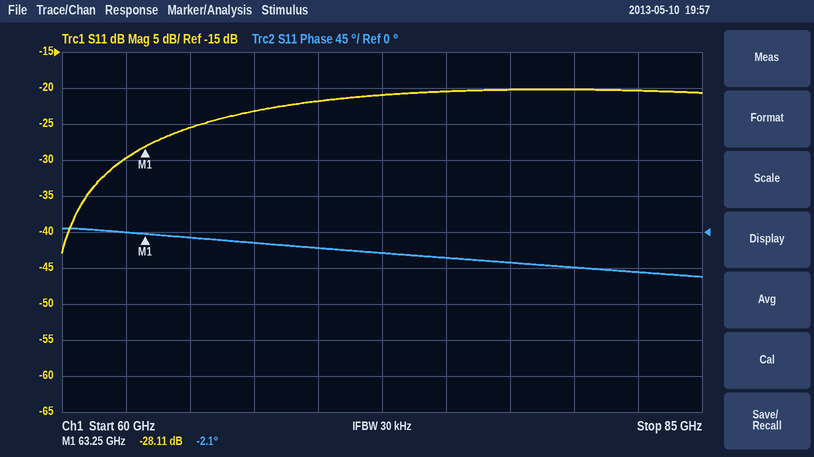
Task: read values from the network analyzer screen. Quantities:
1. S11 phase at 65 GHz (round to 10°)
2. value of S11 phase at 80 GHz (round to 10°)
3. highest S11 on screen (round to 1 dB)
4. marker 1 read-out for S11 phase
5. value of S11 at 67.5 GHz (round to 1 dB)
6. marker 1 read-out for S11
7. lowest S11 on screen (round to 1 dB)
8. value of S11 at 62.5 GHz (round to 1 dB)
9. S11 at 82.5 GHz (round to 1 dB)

-10°
-40°
-20 dB
-2.1°
-23 dB
-28.11 dB
-43 dB
-30 dB
-20 dB
